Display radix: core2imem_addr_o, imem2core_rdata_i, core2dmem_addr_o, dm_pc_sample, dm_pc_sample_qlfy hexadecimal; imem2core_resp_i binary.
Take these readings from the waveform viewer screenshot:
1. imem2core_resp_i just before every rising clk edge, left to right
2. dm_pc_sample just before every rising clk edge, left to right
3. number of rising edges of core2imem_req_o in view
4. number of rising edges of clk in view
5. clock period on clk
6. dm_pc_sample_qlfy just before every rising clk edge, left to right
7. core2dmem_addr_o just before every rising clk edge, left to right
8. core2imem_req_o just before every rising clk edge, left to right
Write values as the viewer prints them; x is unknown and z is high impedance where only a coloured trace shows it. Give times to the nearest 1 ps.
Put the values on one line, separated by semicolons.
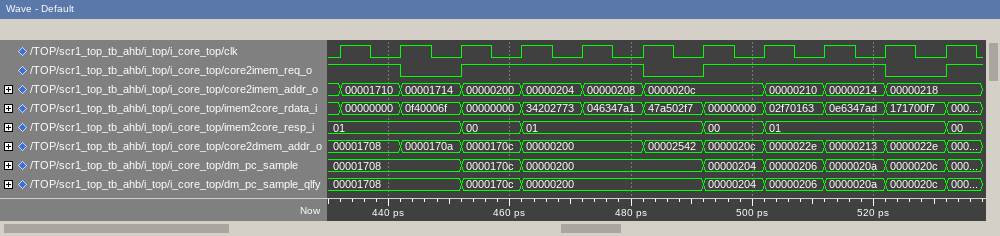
01, 01, 01, 00, 01, 01, 01, 00, 01, 01, 01; 00001708, 00001708, 00001708, 0000170c, 00000200, 00000200, 00000200, 00000204, 00000206, 0000020a, 0000020c; 3; 11; 10 ps; 00001708, 00001708, 00001708, 0000170c, 00000200, 00000200, 00000200, 00000204, 00000206, 0000020a, 0000020c; 00001708, 00001708, 0000170a, 0000170c, 00000200, 00000200, 00002542, 0000020c, 0000022e, 00000213, 0000022e; 1 1 0 1 1 1 0 1 1 1 0
